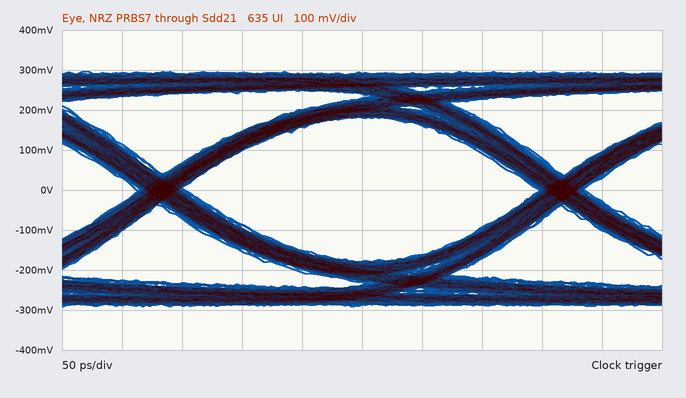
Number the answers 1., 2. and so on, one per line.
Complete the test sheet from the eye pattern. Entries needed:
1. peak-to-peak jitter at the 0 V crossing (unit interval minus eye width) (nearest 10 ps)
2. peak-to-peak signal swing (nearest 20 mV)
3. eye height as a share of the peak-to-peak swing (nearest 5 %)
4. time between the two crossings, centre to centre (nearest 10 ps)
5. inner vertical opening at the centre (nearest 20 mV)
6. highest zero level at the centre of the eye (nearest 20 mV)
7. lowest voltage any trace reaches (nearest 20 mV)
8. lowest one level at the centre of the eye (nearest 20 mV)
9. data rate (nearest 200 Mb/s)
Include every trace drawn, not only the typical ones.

1. 40 ps
2. 580 mV
3. 60 %
4. 330 ps
5. 360 mV
6. -180 mV
7. -300 mV
8. 180 mV
9. 3.0 Gb/s
